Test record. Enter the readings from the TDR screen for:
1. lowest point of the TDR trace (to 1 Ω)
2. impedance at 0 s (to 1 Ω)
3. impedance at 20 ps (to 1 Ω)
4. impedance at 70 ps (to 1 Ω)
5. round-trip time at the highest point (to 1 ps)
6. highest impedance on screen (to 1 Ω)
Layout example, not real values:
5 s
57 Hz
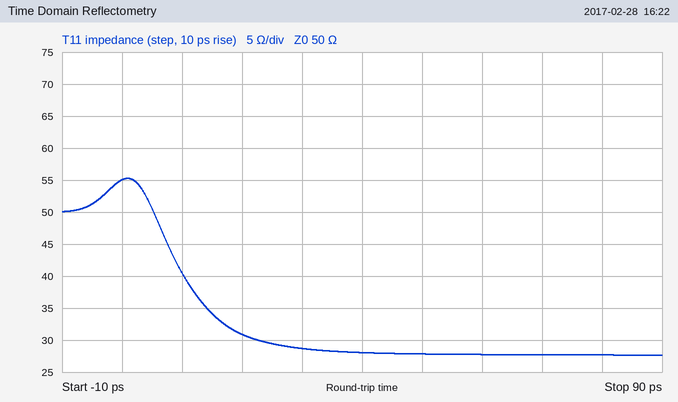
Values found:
28 Ω
55 Ω
31 Ω
28 Ω
1 ps
55 Ω
